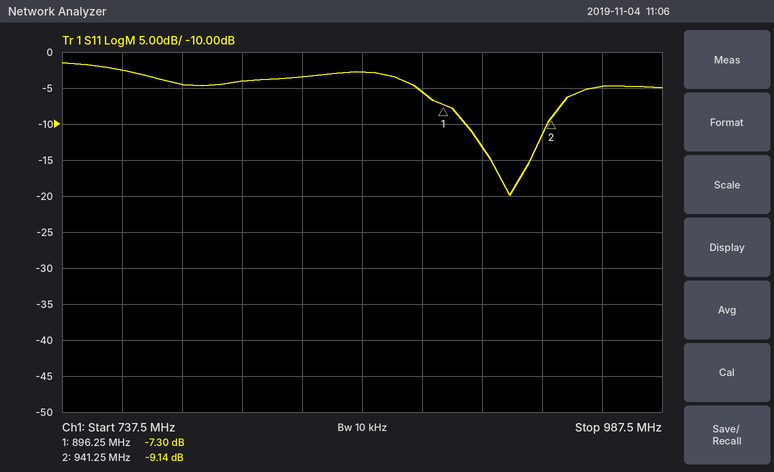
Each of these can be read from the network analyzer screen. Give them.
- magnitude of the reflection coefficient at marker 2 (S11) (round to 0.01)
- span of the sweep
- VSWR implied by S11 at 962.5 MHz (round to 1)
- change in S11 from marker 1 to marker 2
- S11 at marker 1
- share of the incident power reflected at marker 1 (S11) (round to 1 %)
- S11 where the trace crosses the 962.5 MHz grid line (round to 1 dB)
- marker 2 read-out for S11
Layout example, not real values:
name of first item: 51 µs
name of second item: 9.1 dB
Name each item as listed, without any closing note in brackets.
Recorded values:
magnitude of the reflection coefficient at marker 2 (S11): 0.35
span of the sweep: 250 MHz
VSWR implied by S11 at 962.5 MHz: 4
change in S11 from marker 1 to marker 2: -1.84 dB
S11 at marker 1: -7.30 dB
share of the incident power reflected at marker 1 (S11): 19 %
S11 where the trace crosses the 962.5 MHz grid line: -5 dB
marker 2 read-out for S11: -9.14 dB
